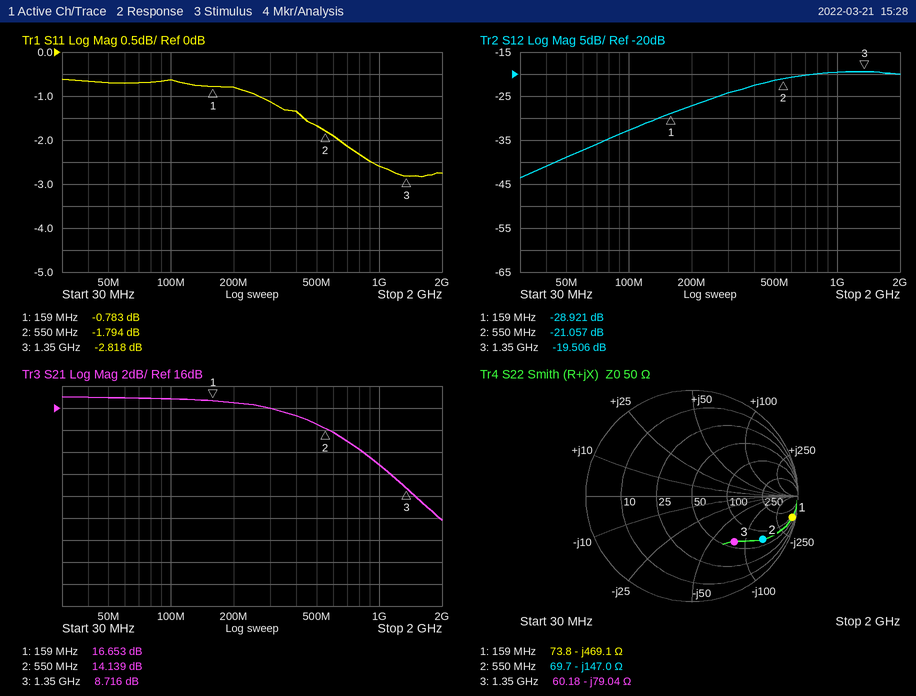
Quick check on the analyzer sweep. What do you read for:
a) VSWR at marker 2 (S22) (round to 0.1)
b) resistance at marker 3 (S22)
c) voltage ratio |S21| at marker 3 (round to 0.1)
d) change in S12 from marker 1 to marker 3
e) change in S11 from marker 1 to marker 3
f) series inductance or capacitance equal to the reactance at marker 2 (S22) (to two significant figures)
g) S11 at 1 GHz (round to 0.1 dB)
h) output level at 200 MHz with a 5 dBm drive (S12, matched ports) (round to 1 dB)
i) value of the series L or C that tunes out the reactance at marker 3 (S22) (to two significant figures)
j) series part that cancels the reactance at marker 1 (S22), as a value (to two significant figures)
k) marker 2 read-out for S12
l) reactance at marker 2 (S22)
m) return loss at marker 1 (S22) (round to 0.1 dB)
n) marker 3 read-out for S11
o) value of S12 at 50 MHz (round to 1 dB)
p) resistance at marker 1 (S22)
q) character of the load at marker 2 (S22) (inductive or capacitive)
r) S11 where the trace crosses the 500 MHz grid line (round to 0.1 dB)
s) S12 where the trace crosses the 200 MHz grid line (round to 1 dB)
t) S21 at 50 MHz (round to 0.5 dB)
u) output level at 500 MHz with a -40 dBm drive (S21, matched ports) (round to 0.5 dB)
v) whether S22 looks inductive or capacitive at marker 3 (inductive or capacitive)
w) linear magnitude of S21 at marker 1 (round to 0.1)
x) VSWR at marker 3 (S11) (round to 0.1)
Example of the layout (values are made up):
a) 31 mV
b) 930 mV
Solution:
a) 8.2
b) 60.18 Ω
c) 2.7
d) 9.415 dB
e) -2.035 dB
f) 2.0 pF
g) -2.6 dB
h) -22 dBm
i) 9.3 nH
j) 470 nH
k) -21.057 dB
l) -147.0 Ω
m) 0.3 dB
n) -2.818 dB
o) -39 dB
p) 73.8 Ω
q) capacitive
r) -1.7 dB
s) -27 dB
t) 17.0 dB
u) -25.5 dBm
v) capacitive
w) 6.8
x) 6.2
